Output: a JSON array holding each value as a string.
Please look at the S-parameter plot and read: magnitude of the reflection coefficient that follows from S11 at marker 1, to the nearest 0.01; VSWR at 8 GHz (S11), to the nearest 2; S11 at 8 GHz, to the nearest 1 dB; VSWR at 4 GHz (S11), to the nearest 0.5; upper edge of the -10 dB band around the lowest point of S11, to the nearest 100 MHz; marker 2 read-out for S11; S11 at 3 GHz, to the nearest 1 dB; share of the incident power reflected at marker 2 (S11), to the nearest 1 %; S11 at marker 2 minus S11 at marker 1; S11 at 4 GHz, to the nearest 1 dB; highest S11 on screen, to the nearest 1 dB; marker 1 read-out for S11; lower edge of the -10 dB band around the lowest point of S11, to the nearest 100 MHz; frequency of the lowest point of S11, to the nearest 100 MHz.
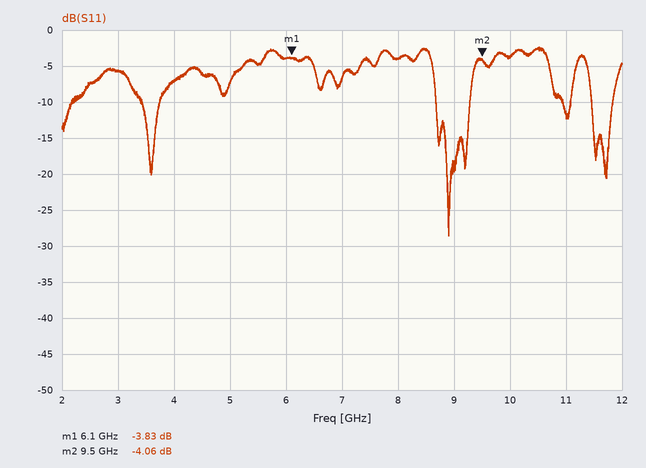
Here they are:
["0.64", "4", "-4 dB", "2.5", "9.3 GHz", "-4.06 dB", "-6 dB", "39 %", "-0.23 dB", "-7 dB", "-2 dB", "-3.83 dB", "8.7 GHz", "8.9 GHz"]
